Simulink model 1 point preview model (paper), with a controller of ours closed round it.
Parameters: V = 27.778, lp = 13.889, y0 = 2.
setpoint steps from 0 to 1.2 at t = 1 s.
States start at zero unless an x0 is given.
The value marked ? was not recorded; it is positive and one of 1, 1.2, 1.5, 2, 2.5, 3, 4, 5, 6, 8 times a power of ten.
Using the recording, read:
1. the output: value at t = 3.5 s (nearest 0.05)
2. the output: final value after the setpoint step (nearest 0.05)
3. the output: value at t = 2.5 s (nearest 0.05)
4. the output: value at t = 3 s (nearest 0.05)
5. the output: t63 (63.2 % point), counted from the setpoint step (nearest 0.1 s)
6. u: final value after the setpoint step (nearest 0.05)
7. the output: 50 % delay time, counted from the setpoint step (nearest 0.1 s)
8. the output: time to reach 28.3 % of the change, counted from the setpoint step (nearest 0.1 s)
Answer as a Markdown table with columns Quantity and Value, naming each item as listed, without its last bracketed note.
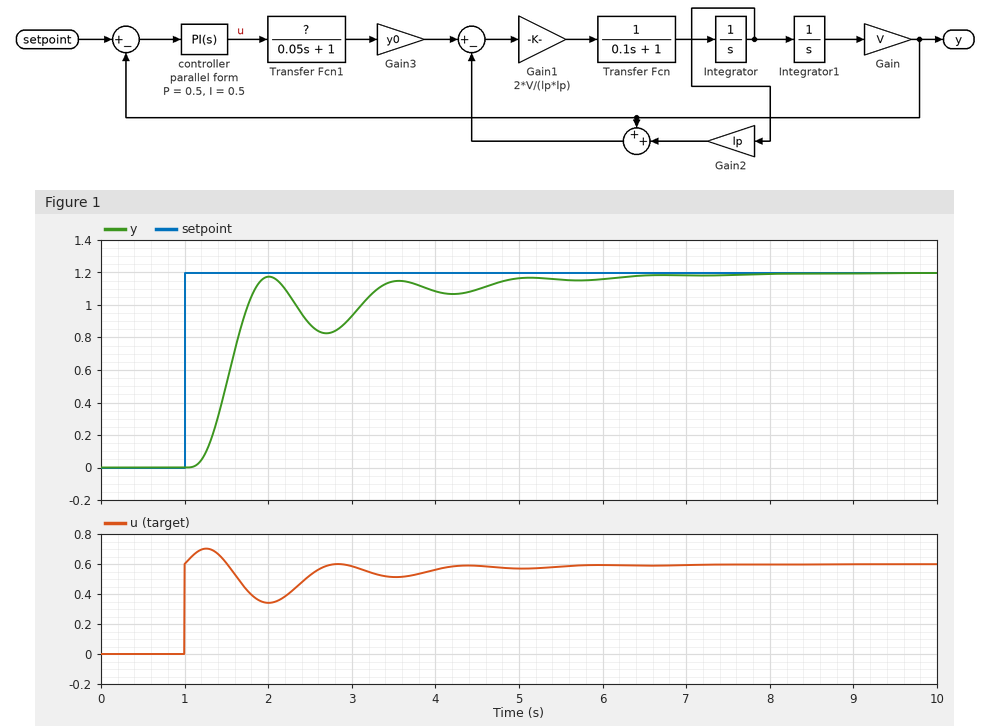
| Quantity | Value |
|---|---|
| the output: value at t = 3.5 s | 1.15 |
| the output: final value after the setpoint step | 1.20 |
| the output: value at t = 2.5 s | 0.90 |
| the output: value at t = 3 s | 0.95 |
| the output: t63 (63.2 % point), counted from the setpoint step | 0.6 s |
| u: final value after the setpoint step | 0.60 |
| the output: 50 % delay time, counted from the setpoint step | 0.5 s |
| the output: time to reach 28.3 % of the change, counted from the setpoint step | 0.4 s |
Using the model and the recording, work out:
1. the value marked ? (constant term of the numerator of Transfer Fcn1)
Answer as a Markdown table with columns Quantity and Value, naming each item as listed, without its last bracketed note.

| Quantity | Value |
|---|---|
| the value marked ? | 1 |
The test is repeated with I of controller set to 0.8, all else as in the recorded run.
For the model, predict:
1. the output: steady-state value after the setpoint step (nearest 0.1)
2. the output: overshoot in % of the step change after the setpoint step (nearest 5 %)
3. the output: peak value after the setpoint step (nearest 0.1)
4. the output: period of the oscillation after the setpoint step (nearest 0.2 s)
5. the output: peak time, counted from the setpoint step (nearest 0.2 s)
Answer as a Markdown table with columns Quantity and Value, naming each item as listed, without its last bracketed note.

| Quantity | Value |
|---|---|
| the output: steady-state value after the setpoint step | 1.2 |
| the output: overshoot in % of the step change after the setpoint step | 15 % |
| the output: peak value after the setpoint step | 1.4 |
| the output: period of the oscillation after the setpoint step | 1.6 s |
| the output: peak time, counted from the setpoint step | 1.0 s |
